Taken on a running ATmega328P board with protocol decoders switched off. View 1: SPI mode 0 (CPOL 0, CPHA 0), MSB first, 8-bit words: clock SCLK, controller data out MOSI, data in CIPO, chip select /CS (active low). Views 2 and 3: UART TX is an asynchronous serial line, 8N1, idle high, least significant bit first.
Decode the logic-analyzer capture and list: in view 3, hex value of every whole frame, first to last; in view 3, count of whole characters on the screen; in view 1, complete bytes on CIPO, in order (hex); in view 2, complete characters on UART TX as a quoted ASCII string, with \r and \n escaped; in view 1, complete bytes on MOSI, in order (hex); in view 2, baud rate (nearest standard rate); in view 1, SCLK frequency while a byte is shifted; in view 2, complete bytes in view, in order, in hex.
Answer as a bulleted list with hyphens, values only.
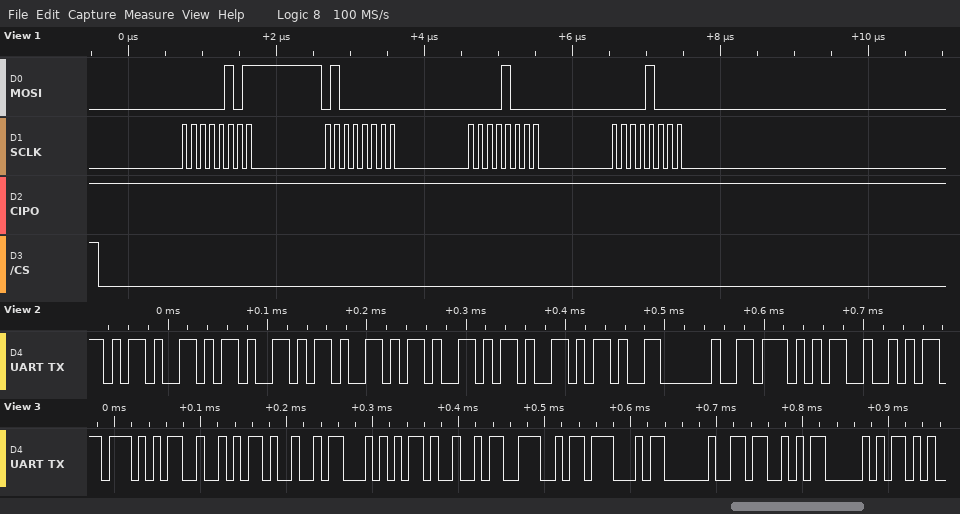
- 57 52 49 54 49 4E 47 20 53 50
- 10
- FF FF FF FF
- "------ WR"
- 05 40 08 08
- 115200 baud
- 8 MHz
- 2D 2D 2D 2D 2D 2D 20 57 52
